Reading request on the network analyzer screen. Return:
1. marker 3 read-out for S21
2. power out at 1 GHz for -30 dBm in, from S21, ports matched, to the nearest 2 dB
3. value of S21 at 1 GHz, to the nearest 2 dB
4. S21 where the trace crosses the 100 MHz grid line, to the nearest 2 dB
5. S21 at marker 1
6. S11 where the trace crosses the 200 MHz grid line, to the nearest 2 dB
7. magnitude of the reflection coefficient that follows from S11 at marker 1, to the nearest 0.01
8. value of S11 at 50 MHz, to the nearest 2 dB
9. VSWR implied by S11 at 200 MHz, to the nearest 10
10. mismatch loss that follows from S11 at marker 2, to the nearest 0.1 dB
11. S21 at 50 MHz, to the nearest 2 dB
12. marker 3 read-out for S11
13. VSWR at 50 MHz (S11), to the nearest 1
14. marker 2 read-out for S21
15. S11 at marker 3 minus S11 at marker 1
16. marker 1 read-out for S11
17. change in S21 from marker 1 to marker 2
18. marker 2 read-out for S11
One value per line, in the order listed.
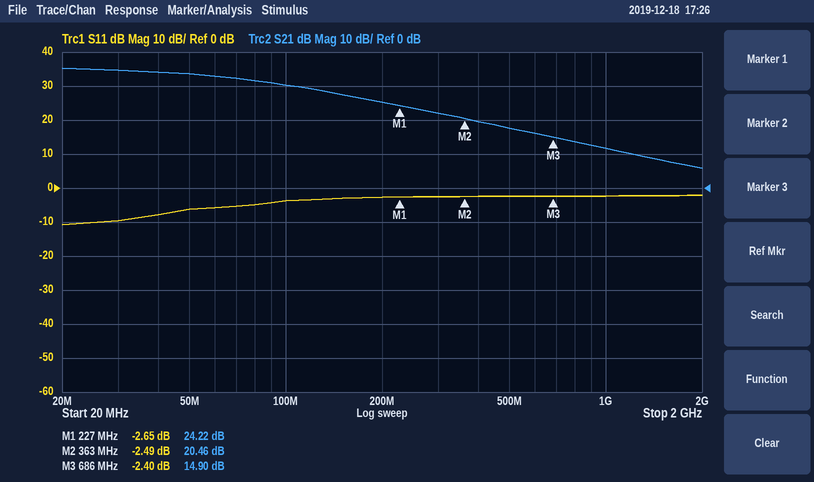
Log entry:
14.90 dB
-18 dBm
12 dB
30 dB
24.22 dB
-2 dB
0.74
-6 dB
10
3.6 dB
34 dB
-2.40 dB
3
20.46 dB
0.25 dB
-2.65 dB
-3.76 dB
-2.49 dB
